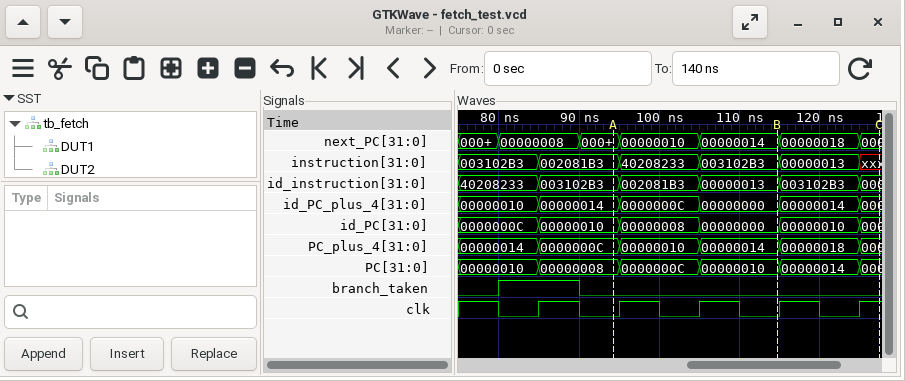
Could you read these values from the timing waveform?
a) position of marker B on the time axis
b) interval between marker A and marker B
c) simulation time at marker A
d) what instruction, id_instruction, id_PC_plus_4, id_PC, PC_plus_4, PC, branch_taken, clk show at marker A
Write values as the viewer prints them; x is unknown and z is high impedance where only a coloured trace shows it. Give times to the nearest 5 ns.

115 ns
20 ns
95 ns
instruction=002081B3, id_instruction=003102B3, id_PC_plus_4=00000014, id_PC=00000010, PC_plus_4=0000000C, PC=00000008, branch_taken=0, clk=0
